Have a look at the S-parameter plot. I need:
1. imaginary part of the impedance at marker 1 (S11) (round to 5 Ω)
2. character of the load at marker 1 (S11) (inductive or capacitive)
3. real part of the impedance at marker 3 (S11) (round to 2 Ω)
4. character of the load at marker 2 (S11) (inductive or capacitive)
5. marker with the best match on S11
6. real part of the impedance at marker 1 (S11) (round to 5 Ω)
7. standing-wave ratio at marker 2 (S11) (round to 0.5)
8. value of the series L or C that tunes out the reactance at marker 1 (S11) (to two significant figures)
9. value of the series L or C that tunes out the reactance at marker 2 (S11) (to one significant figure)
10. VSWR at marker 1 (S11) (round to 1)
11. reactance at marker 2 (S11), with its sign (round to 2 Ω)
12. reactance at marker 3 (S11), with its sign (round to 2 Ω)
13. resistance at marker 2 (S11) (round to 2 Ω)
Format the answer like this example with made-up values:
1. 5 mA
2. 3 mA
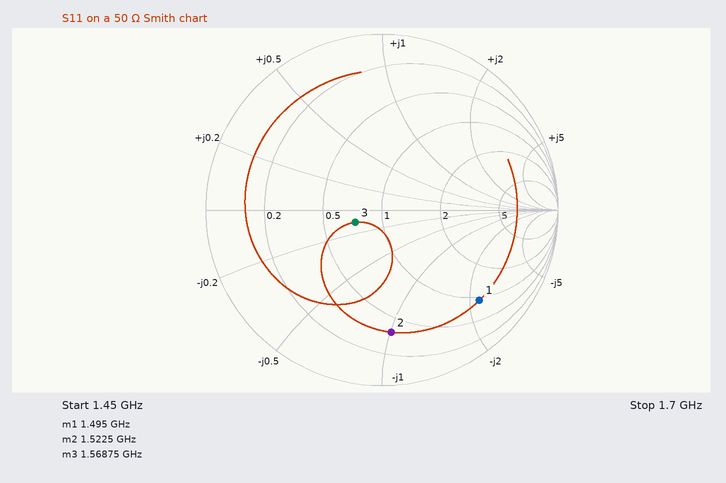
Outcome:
1. -110 Ω
2. capacitive
3. 36 Ω
4. capacitive
5. marker 3
6. 45 Ω
7. 5.5
8. 12 nH
9. 5 nH
10. 7
11. -50 Ω
12. -6 Ω
13. 18 Ω
